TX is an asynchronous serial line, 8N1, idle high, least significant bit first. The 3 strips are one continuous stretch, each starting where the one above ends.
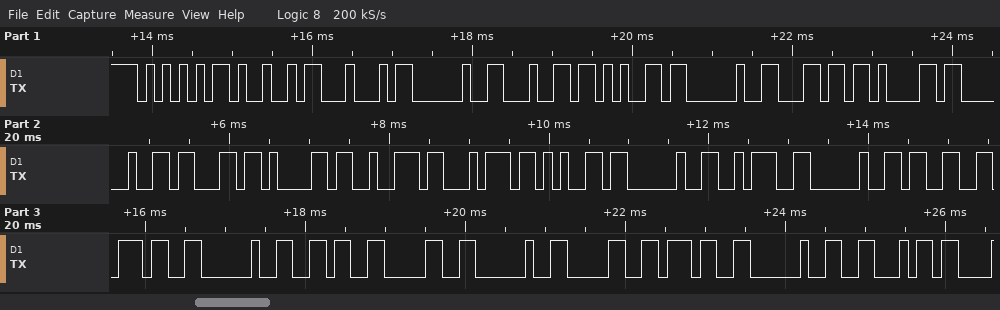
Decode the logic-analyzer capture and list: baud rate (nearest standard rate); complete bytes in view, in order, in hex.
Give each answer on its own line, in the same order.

9600 baud
55 49 44 20 64 65 20 6C 61 20 63 61 72 74 65 20 3A 20 33 37 20 36 30 20 30 37 20 46
